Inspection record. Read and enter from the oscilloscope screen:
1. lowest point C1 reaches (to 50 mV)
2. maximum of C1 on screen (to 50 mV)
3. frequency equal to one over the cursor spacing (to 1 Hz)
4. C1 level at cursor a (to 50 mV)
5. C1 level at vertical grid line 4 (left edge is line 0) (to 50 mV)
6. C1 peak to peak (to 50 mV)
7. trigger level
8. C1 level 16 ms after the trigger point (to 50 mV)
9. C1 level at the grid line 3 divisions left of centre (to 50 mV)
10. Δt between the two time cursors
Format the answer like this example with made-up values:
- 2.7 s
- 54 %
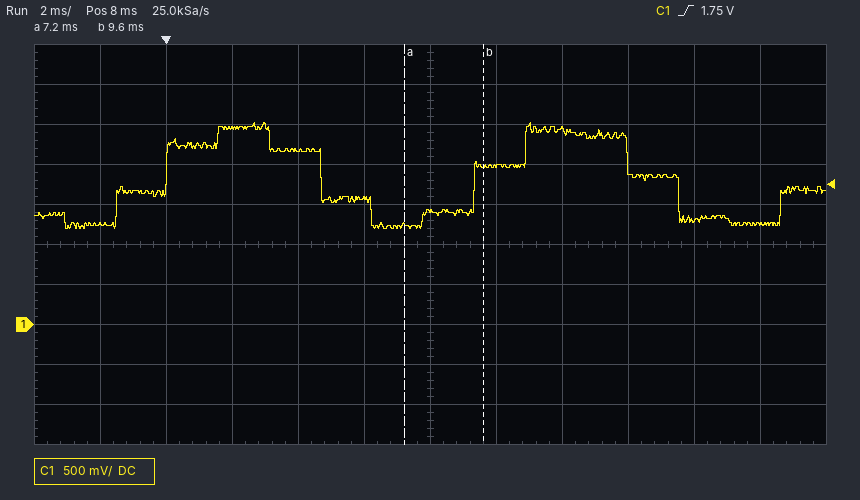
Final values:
- 1.20 V
- 2.50 V
- 417 Hz
- 1.25 V
- 2.20 V
- 1.30 V
- 1.75 V
- 1.30 V
- 2.45 V
- 2.4 ms
